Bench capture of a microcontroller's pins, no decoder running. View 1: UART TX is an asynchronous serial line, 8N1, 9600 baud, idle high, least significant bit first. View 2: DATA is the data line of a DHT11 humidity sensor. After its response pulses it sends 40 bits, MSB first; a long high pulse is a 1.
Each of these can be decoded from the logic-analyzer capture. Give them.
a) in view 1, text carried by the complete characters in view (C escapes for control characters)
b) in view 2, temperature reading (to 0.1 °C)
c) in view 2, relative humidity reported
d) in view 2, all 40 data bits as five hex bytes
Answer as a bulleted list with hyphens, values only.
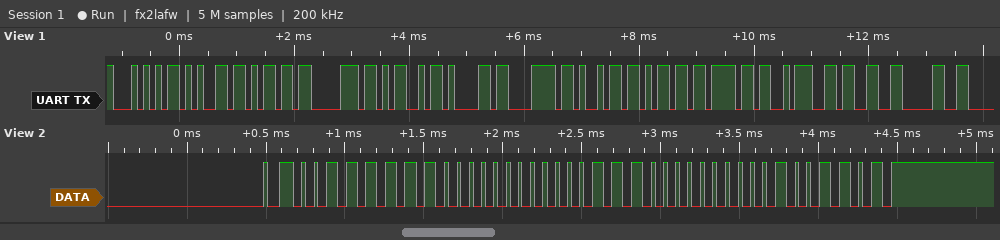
- "TempMaximo:30"
- 14.0 °C
- 63 %
- 3F 00 0E 00 4D
